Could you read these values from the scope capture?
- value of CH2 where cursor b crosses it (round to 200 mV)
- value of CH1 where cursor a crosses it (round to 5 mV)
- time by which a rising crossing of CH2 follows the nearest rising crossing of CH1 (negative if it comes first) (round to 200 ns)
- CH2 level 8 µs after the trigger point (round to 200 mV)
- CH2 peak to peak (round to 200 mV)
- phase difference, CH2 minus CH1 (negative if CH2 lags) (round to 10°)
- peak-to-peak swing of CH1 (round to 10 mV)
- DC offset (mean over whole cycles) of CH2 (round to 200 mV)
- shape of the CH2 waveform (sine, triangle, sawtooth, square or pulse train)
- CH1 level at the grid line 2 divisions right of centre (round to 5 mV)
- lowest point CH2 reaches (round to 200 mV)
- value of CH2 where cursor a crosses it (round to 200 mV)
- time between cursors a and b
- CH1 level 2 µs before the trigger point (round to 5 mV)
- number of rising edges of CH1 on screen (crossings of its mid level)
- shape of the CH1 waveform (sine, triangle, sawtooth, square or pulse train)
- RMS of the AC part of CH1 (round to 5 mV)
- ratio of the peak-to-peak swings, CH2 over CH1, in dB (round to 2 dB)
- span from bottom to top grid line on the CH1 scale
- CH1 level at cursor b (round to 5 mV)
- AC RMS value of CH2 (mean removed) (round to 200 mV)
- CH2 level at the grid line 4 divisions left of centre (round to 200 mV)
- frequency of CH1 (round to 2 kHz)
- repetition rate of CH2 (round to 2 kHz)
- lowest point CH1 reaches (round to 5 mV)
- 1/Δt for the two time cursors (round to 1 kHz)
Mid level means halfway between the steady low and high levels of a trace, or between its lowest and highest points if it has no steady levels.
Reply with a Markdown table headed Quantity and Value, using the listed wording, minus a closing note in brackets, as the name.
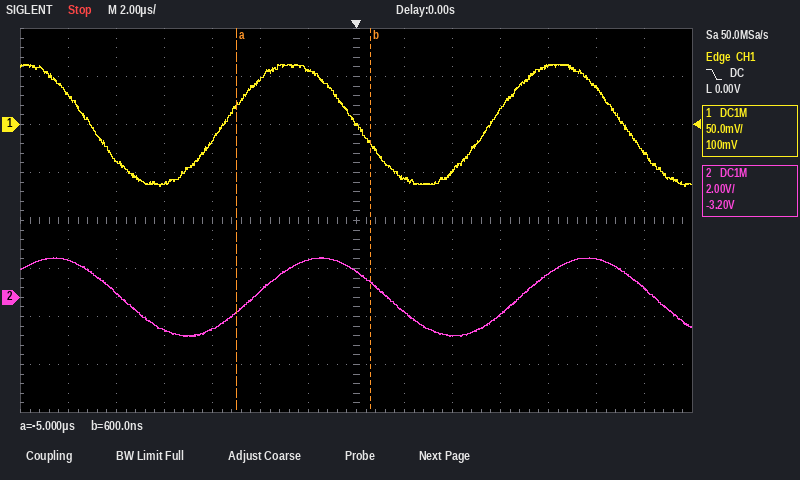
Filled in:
| Quantity | Value |
|---|---|
| value of CH2 where cursor b crosses it | 600 mV |
| value of CH1 where cursor a crosses it | 20 mV |
| time by which a rising crossing of CH2 follows the nearest rising crossing of CH1 (negative if it comes first) | +1.2 µs |
| CH2 level 8 µs after the trigger point | 1.0 V |
| CH2 peak to peak | 3.2 V |
| phase difference, CH2 minus CH1 (negative if CH2 lags) | -40° |
| peak-to-peak swing of CH1 | 130 mV |
| DC offset (mean over whole cycles) of CH2 | 0.0 V |
| shape of the CH2 waveform | sine |
| CH1 level at the grid line 2 divisions right of centre | -50 mV |
| lowest point CH2 reaches | -1.6 V |
| value of CH2 where cursor a crosses it | -600 mV |
| time between cursors a and b | 5.6 µs |
| CH1 level 2 µs before the trigger point | 55 mV |
| number of rising edges of CH1 on screen | 2 |
| shape of the CH1 waveform | sine |
| RMS of the AC part of CH1 | 45 mV |
| ratio of the peak-to-peak swings, CH2 over CH1, in dB | 28 dB |
| span from bottom to top grid line on the CH1 scale | 400 mV |
| CH1 level at cursor b | -20 mV |
| AC RMS value of CH2 (mean removed) | 1.2 V |
| CH2 level at the grid line 4 divisions left of centre | -1.4 V |
| frequency of CH1 | 90 kHz |
| repetition rate of CH2 | 90 kHz |
| lowest point CH1 reaches | -65 mV |
| 1/Δt for the two time cursors | 179 kHz |
